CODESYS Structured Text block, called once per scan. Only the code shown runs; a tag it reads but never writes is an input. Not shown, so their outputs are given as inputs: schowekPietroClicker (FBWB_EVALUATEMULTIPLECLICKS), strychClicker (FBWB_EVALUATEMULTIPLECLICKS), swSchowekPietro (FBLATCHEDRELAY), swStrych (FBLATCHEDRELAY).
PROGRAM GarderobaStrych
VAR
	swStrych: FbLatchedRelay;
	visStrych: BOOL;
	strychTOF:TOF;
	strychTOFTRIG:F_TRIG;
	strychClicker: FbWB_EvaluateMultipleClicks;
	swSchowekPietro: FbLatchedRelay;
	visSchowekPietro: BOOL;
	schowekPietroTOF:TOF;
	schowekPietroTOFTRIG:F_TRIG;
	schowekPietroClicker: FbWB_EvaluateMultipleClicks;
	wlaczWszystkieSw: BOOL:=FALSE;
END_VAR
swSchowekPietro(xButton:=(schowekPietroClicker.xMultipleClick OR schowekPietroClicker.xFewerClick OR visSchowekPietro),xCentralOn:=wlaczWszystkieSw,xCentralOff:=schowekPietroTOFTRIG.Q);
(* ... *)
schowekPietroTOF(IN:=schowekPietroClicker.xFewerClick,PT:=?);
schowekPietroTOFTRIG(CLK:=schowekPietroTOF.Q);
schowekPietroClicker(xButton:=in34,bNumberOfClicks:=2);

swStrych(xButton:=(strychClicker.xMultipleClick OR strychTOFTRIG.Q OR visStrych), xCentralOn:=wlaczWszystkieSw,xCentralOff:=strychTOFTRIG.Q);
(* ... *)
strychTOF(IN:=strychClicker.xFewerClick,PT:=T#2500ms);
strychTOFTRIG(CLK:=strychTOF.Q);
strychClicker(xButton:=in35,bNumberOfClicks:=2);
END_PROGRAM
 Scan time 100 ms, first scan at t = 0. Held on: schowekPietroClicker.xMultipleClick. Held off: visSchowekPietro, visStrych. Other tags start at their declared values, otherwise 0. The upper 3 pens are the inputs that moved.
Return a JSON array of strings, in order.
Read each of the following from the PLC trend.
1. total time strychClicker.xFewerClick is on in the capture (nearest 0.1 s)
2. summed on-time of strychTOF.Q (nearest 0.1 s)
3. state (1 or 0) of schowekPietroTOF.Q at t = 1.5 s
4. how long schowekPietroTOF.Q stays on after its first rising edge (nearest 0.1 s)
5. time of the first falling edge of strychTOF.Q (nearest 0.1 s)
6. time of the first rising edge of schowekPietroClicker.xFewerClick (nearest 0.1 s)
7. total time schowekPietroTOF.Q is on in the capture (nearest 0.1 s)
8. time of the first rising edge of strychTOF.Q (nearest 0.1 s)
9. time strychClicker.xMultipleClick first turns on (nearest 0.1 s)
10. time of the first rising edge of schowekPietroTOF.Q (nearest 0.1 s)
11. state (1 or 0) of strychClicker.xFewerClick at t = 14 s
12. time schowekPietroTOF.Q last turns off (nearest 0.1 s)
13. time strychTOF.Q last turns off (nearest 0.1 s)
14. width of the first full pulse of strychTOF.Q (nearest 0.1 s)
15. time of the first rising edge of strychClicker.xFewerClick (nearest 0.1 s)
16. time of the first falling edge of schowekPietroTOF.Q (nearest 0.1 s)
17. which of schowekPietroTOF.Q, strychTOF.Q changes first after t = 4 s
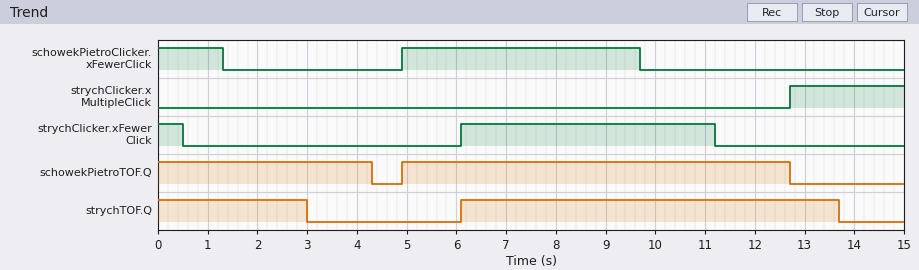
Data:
["5.6 s", "10.6 s", "1", "7.8 s", "3.0 s", "4.9 s", "12.1 s", "6.1 s", "12.7 s", "4.9 s", "0", "12.7 s", "13.7 s", "7.6 s", "6.1 s", "4.3 s", "schowekPietroTOF.Q"]
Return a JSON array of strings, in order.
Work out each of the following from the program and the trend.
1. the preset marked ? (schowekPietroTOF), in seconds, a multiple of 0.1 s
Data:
["3.0 s"]
